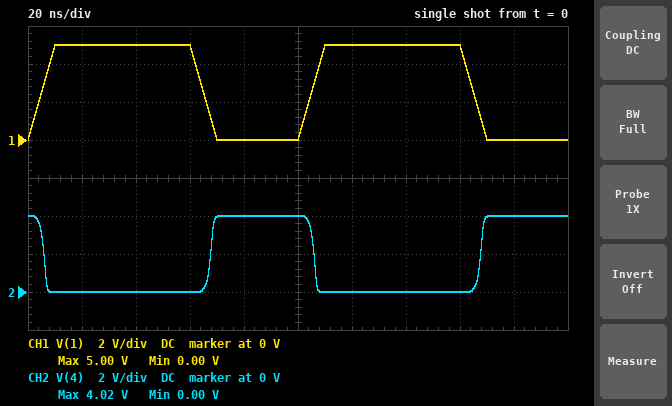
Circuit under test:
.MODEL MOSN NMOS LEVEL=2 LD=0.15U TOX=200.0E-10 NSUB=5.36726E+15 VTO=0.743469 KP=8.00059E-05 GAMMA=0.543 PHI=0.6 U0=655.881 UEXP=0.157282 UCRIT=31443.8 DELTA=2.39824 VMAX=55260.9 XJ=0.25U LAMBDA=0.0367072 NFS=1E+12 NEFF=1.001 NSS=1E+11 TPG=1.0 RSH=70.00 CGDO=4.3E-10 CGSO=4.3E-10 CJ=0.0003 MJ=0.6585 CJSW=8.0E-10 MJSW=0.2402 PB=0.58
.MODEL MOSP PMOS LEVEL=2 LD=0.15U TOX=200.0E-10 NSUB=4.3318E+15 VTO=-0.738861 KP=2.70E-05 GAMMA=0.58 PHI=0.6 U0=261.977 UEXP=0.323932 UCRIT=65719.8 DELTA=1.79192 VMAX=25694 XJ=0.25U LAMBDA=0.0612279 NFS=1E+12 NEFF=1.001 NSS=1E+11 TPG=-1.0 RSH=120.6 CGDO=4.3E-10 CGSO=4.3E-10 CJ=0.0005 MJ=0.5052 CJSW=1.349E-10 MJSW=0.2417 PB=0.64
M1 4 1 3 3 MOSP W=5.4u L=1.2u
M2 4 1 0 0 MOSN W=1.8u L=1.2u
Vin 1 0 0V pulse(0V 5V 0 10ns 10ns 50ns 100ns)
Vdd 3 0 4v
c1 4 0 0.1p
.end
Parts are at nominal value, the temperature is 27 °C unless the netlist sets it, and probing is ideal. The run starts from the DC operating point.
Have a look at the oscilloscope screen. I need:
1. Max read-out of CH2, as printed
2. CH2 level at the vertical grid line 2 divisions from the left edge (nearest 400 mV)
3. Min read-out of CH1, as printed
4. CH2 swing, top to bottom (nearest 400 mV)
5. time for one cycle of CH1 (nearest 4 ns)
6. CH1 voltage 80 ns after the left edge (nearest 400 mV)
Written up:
4.02 V
0 V
0.00 V
4.0 V
100 ns
0 V
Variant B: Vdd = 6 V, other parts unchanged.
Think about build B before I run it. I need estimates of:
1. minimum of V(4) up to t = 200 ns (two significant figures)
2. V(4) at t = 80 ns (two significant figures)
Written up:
56 mV
6.0 V
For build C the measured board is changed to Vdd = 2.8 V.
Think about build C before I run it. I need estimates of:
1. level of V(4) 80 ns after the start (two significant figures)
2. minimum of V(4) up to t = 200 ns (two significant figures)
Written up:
2.8 V
-11 mV
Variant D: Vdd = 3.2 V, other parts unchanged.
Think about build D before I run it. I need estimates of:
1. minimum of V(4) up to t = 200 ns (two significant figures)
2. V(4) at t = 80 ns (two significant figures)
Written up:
-9.6 mV
3.2 V
